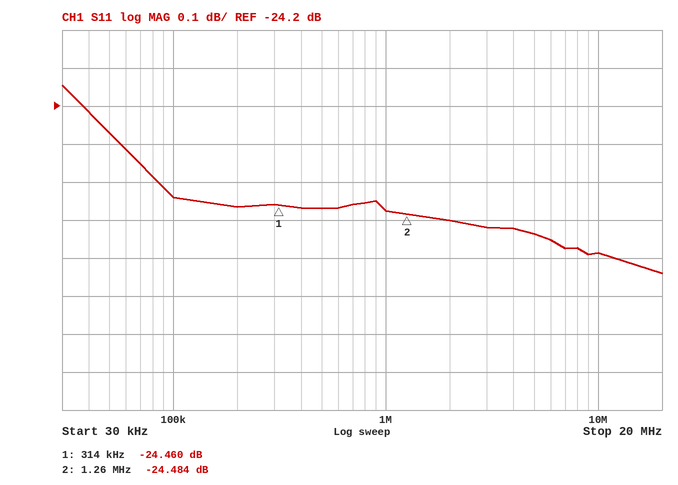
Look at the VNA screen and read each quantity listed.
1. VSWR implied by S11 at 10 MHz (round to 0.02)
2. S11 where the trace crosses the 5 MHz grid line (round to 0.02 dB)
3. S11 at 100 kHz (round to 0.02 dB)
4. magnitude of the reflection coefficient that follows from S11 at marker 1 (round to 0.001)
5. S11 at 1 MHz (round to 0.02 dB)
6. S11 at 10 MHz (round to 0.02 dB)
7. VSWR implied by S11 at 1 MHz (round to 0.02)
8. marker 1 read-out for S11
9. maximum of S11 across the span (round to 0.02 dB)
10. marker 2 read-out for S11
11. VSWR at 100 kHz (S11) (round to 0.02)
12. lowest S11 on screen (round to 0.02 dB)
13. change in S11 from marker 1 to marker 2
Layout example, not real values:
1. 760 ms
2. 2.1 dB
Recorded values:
1. 1.12
2. -24.54 dB
3. -24.44 dB
4. 0.060
5. -24.48 dB
6. -24.58 dB
7. 1.12
8. -24.460 dB
9. -24.14 dB
10. -24.484 dB
11. 1.12
12. -24.64 dB
13. -0.024 dB
